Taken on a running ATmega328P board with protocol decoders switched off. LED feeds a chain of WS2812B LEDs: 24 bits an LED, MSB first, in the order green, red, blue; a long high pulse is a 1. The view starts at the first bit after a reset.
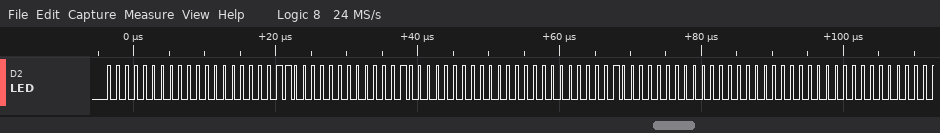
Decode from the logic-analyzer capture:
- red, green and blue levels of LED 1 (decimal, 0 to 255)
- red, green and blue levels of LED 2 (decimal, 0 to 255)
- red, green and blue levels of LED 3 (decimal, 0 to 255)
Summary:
0, 0, 24
64, 0, 0
64, 0, 0
